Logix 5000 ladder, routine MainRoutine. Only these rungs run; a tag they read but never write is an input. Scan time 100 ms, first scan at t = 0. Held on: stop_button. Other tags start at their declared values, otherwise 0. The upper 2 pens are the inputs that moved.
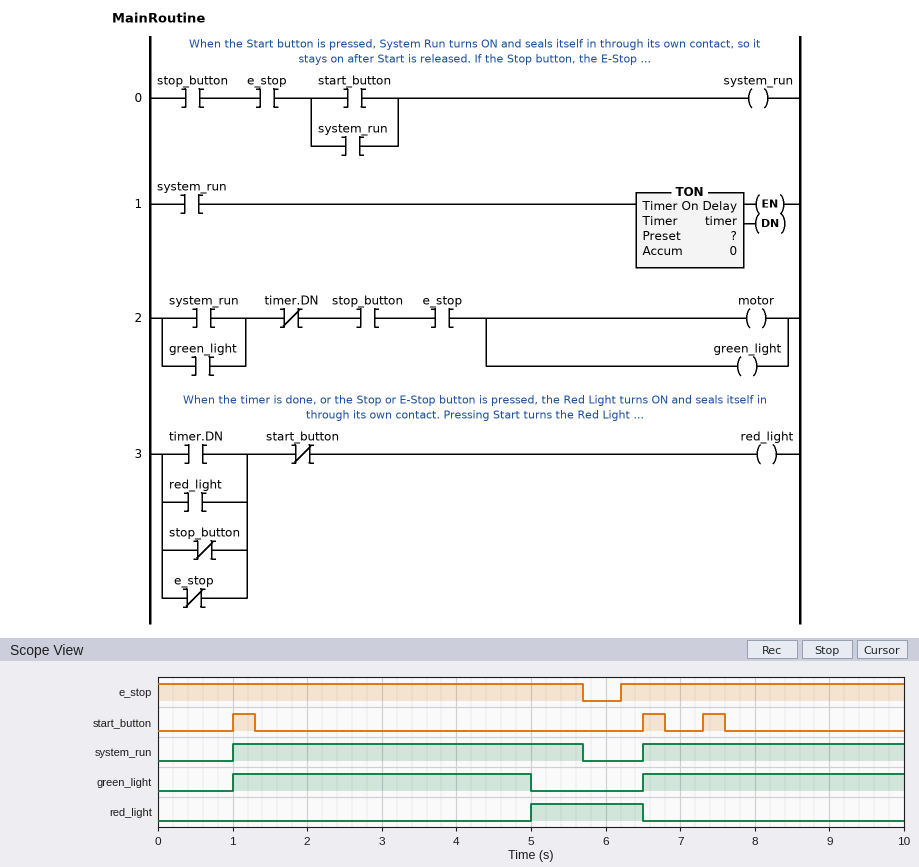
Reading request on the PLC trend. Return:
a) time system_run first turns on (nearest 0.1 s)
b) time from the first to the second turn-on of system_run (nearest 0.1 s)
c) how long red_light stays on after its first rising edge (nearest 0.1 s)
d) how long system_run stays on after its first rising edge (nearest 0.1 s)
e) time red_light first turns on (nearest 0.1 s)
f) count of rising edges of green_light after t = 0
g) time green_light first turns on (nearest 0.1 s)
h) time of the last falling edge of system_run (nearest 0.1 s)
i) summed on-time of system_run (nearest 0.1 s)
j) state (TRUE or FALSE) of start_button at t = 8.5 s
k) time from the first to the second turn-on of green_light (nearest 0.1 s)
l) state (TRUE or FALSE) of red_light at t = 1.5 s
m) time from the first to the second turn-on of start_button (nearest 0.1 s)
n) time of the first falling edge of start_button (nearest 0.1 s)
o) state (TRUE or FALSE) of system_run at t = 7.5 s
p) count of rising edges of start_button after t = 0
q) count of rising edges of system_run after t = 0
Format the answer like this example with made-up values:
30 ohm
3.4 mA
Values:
1.0 s
5.5 s
1.5 s
4.7 s
5.0 s
2
1.0 s
5.7 s
8.2 s
FALSE
5.5 s
FALSE
5.5 s
1.3 s
TRUE
3
2
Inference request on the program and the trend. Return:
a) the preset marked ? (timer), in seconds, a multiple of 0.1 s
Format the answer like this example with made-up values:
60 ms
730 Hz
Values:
4.0 s
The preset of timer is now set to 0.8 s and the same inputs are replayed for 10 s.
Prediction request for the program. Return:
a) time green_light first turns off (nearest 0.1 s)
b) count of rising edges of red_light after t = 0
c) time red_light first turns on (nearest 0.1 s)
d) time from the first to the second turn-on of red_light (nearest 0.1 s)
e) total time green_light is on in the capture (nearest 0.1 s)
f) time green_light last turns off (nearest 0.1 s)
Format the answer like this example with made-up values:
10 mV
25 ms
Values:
1.8 s
2
1.8 s
5.8 s
1.6 s
7.3 s
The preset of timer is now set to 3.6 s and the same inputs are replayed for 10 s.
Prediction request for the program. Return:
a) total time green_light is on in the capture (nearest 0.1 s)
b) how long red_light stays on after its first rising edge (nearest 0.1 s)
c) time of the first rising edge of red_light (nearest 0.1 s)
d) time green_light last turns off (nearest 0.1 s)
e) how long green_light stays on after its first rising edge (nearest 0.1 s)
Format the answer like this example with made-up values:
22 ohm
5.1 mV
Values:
7.1 s
1.9 s
4.6 s
4.6 s
3.6 s
